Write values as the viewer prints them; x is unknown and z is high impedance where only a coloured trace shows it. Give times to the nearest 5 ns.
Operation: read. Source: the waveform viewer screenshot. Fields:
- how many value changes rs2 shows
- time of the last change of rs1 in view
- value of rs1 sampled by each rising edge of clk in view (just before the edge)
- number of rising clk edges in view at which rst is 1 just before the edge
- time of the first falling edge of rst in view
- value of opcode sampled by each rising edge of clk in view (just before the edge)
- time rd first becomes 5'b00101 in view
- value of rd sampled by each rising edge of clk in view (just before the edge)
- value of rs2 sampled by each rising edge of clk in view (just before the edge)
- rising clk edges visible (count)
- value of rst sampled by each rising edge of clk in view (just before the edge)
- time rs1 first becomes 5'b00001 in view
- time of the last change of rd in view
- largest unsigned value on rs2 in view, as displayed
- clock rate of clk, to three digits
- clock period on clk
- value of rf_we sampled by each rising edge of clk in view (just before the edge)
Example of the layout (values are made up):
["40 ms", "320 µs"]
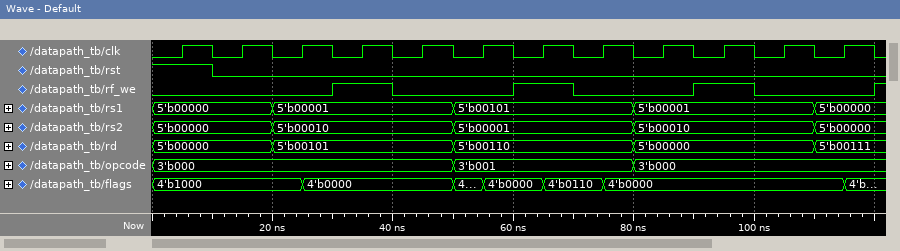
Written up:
["4", "110 ns", "5'b00000, 5'b00000, 5'b00001, 5'b00001, 5'b00001, 5'b00101, 5'b00101, 5'b00101, 5'b00001, 5'b00001, 5'b00001, 5'b00000", "1", "10 ns", "3'b000, 3'b000, 3'b000, 3'b000, 3'b000, 3'b001, 3'b001, 3'b001, 3'b000, 3'b000, 3'b000, 3'b000", "20 ns", "5'b00000, 5'b00000, 5'b00101, 5'b00101, 5'b00101, 5'b00110, 5'b00110, 5'b00110, 5'b00000, 5'b00000, 5'b00000, 5'b00111", "5'b00000, 5'b00000, 5'b00010, 5'b00010, 5'b00010, 5'b00001, 5'b00001, 5'b00001, 5'b00010, 5'b00010, 5'b00010, 5'b00000", "12", "1 0 0 0 0 0 0 0 0 0 0 0", "20 ns", "110 ns", "5'b00010", "100 MHz", "10 ns", "0 0 0 1 0 0 1 0 0 1 0 0"]
